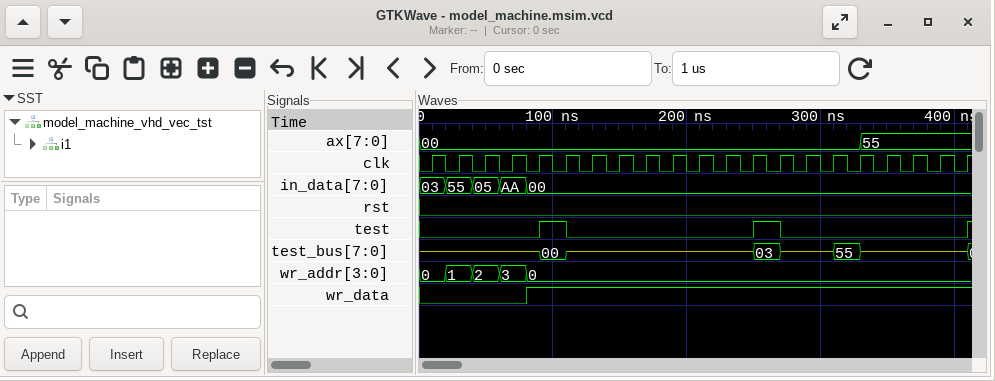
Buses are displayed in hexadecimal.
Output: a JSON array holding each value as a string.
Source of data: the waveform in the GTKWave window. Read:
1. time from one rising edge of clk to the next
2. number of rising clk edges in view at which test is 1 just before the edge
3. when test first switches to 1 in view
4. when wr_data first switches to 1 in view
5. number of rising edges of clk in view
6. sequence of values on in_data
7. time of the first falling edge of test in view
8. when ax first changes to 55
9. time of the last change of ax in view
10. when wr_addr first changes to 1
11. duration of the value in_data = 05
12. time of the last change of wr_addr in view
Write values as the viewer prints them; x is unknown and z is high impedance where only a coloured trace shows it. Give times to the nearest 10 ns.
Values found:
["20 ns", "2", "90 ns", "80 ns", "21", "03, 55, 05, AA, 00", "110 ns", "330 ns", "330 ns", "20 ns", "20 ns", "80 ns"]
